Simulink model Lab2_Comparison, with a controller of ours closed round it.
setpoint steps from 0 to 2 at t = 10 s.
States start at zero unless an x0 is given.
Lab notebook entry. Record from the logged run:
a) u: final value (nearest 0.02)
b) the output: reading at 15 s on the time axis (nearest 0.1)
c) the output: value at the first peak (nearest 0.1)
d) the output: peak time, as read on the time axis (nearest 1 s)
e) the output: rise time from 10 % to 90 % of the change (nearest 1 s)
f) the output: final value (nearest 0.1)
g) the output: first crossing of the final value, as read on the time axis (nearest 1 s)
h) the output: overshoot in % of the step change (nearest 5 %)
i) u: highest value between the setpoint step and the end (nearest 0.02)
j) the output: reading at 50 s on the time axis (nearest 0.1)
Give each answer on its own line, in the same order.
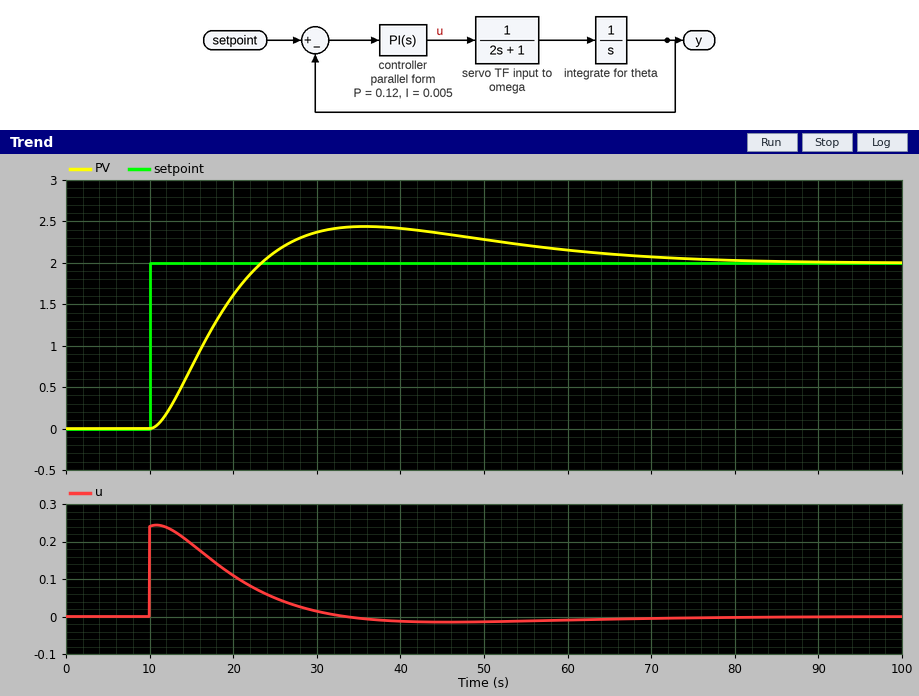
0.00
0.7
2.4
36 s
9 s
2.0
23 s
20 %
0.24
2.3
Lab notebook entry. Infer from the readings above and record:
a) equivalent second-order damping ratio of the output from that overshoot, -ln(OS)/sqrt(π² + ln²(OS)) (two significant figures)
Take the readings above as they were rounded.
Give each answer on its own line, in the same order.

0.46
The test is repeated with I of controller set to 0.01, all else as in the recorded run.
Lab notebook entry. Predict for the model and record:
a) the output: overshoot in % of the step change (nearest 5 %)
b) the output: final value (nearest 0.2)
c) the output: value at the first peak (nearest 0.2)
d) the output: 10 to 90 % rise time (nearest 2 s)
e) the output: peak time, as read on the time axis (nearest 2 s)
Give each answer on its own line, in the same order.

35 %
2.0
2.8
8 s
32 s
